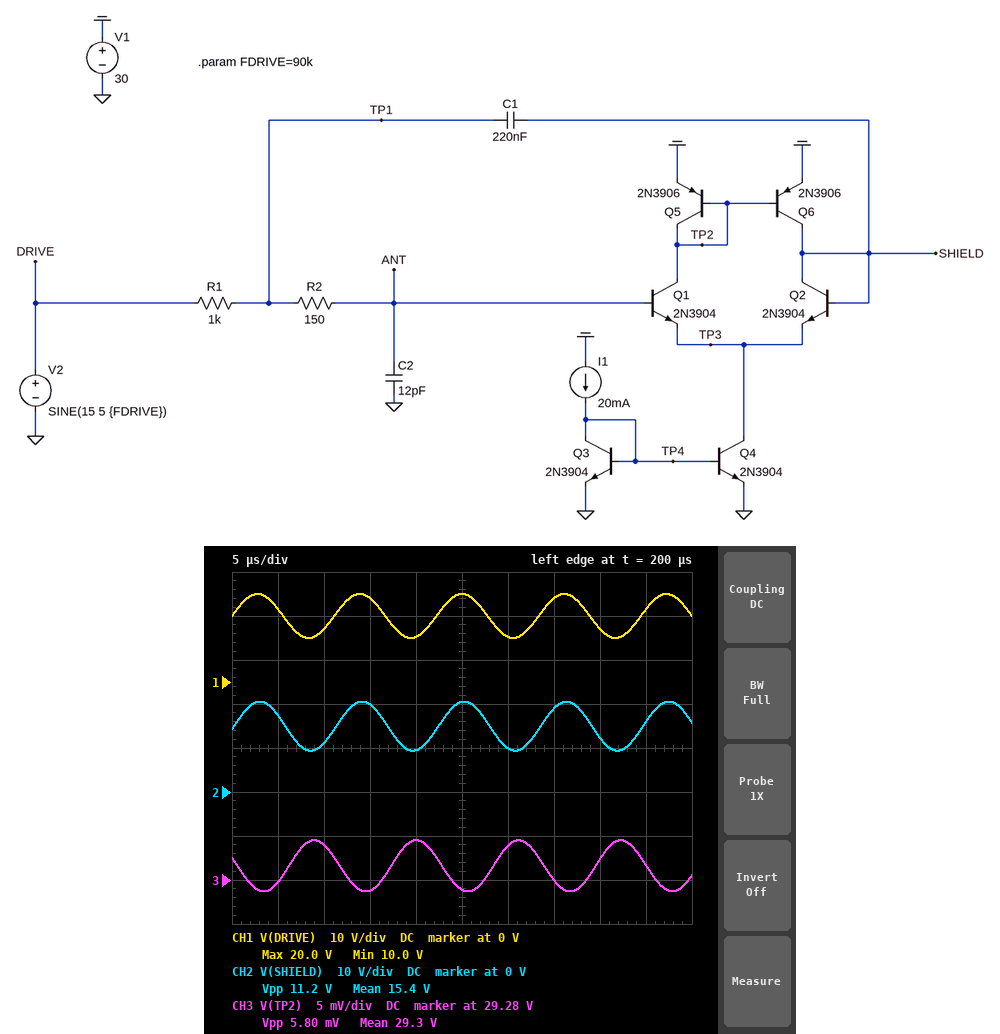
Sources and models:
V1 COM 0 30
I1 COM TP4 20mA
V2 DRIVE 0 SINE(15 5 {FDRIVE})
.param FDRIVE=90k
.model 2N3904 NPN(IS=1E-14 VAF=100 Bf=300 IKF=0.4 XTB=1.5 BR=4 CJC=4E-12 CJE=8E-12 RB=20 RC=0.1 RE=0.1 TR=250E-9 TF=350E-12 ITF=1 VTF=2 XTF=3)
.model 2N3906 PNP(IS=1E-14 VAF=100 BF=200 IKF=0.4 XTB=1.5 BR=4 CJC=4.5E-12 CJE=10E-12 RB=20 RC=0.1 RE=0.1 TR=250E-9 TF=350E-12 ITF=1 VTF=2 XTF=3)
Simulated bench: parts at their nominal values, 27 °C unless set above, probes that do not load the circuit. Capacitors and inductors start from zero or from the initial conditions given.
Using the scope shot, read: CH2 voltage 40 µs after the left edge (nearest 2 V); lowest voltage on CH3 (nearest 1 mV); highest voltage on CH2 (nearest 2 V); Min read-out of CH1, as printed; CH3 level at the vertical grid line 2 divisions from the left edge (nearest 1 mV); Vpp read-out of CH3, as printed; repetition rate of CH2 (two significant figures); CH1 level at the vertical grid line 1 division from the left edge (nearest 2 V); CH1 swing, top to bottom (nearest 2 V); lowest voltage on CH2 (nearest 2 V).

12 V
29.279 V
20 V
10.0 V
29.284 V
5.80 mV
90 kHz
16 V
10 V
10 V
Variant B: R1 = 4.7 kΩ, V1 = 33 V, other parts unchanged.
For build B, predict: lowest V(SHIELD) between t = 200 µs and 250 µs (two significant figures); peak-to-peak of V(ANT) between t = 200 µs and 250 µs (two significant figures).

7.8 V
14 V
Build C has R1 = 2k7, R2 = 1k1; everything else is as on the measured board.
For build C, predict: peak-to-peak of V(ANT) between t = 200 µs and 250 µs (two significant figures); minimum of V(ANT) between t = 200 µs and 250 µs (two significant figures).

5.3 V
12 V
